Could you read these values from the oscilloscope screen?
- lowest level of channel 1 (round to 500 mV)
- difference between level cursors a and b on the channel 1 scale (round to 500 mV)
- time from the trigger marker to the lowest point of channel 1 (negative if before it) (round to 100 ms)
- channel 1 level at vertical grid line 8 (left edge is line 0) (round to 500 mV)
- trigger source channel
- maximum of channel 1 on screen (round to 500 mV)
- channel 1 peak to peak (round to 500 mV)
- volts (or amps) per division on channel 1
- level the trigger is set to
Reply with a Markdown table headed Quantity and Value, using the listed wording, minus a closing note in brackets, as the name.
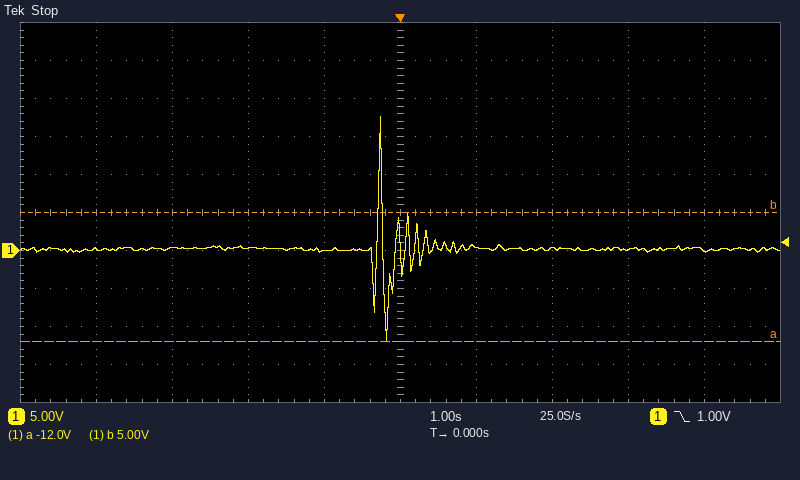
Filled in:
| Quantity | Value |
|---|---|
| lowest level of channel 1 | -12.0 V |
| difference between level cursors a and b on the channel 1 scale | 17.0 V |
| time from the trigger marker to the lowest point of channel 1 (negative if before it) | -200 ms |
| channel 1 level at vertical grid line 8 (left edge is line 0) | 0.0 V |
| trigger source channel | channel 1 |
| maximum of channel 1 on screen | 17.5 V |
| channel 1 peak to peak | 29.5 V |
| volts (or amps) per division on channel 1 | 5 V |
| level the trigger is set to | 1.00 V |
